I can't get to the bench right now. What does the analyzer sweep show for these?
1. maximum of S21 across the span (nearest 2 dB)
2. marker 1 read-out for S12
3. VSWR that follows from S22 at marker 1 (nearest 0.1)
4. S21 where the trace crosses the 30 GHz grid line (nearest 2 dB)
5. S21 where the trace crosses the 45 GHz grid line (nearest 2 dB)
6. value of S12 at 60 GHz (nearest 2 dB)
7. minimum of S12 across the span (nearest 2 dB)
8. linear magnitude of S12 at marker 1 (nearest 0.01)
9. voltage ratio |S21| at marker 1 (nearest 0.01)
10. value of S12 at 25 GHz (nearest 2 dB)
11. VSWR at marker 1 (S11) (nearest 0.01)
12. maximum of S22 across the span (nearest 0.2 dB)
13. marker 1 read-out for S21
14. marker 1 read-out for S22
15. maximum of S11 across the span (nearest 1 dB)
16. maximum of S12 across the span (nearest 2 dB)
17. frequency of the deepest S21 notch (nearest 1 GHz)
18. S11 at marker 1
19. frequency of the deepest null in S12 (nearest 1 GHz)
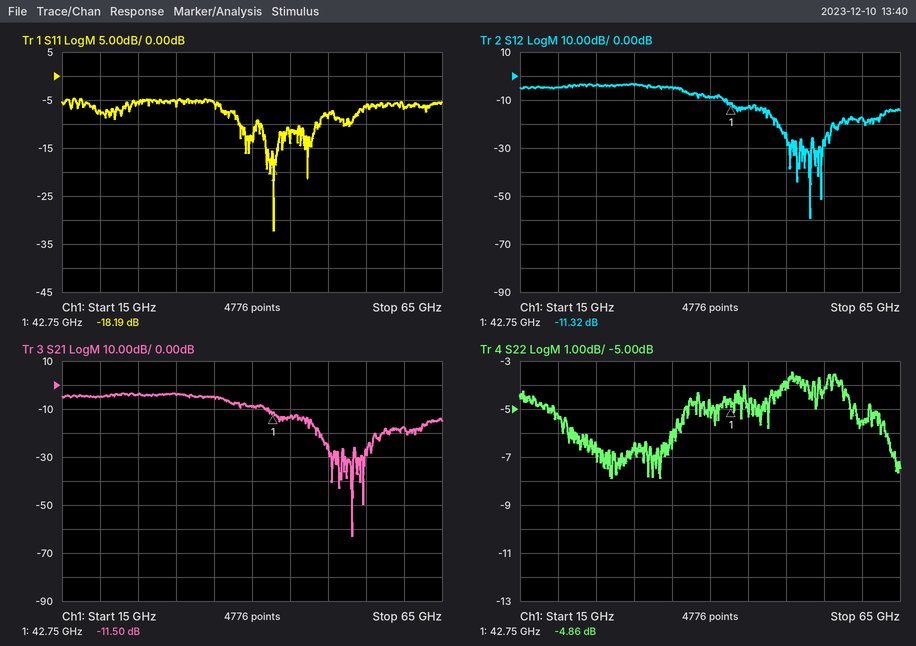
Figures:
-4 dB
-11.32 dB
3.7
-4 dB
-14 dB
-18 dB
-60 dB
0.27
0.27
-4 dB
1.28
-3.4 dB
-11.50 dB
-4.86 dB
-5 dB
-4 dB
53 GHz
-18.19 dB
53 GHz
